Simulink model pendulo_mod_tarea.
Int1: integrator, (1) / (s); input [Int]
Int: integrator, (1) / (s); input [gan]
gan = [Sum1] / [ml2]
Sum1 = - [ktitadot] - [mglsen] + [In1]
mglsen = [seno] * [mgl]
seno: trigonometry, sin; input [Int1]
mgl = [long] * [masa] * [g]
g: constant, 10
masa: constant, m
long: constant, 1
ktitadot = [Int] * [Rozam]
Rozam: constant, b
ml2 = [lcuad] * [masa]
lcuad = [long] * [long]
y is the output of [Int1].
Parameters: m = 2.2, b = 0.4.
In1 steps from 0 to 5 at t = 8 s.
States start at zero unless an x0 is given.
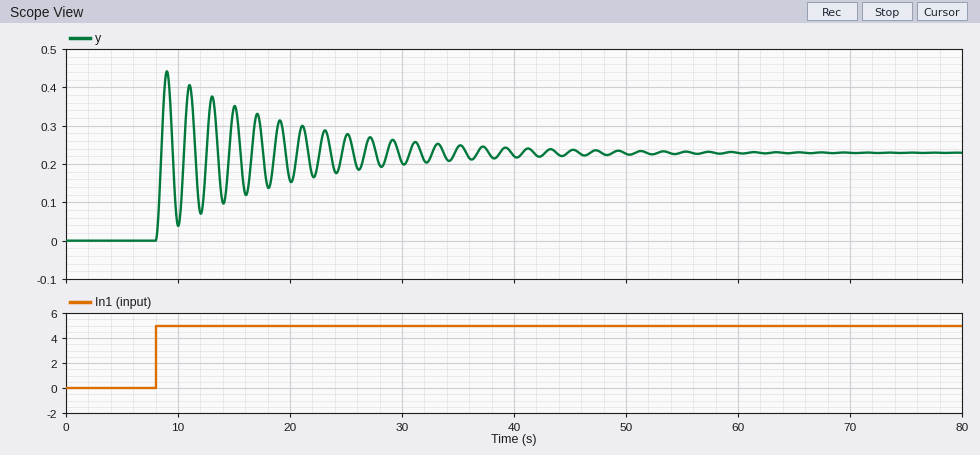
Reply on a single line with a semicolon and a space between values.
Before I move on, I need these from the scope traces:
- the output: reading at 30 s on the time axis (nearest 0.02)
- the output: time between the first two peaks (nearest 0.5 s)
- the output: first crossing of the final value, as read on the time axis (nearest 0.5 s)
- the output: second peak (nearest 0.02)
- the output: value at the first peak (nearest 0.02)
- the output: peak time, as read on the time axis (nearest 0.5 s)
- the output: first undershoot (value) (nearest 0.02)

0.20; 2.0 s; 8.5 s; 0.40; 0.44; 9.0 s; 0.04
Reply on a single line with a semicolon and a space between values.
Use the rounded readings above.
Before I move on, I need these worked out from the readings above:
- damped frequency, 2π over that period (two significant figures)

3.1 rad/s
